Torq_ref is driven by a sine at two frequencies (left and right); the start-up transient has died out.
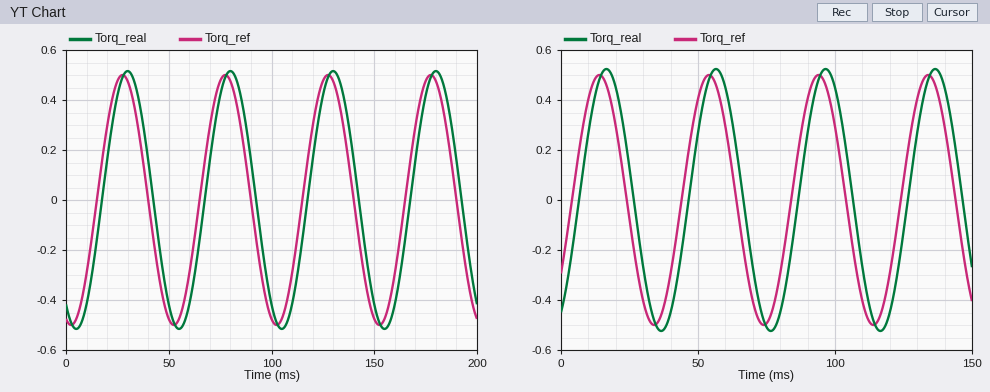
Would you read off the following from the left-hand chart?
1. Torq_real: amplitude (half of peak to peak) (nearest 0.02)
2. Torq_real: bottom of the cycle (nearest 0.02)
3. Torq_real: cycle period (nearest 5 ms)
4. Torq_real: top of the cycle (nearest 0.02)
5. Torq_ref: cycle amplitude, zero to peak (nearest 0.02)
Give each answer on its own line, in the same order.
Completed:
0.52
-0.52
50 ms
0.52
0.50
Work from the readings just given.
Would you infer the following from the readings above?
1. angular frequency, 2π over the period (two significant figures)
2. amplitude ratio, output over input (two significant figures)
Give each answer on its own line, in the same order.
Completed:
0.13 rad/ms
1.0
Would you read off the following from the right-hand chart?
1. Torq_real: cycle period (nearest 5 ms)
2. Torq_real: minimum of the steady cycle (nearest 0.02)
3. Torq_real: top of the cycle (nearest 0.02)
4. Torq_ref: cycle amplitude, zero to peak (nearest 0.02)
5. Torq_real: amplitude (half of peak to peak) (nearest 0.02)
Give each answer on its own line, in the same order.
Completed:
40 ms
-0.52
0.52
0.50
0.52
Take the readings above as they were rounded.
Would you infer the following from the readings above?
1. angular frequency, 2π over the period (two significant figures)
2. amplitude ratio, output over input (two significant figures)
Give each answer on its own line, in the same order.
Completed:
0.16 rad/ms
1.0
